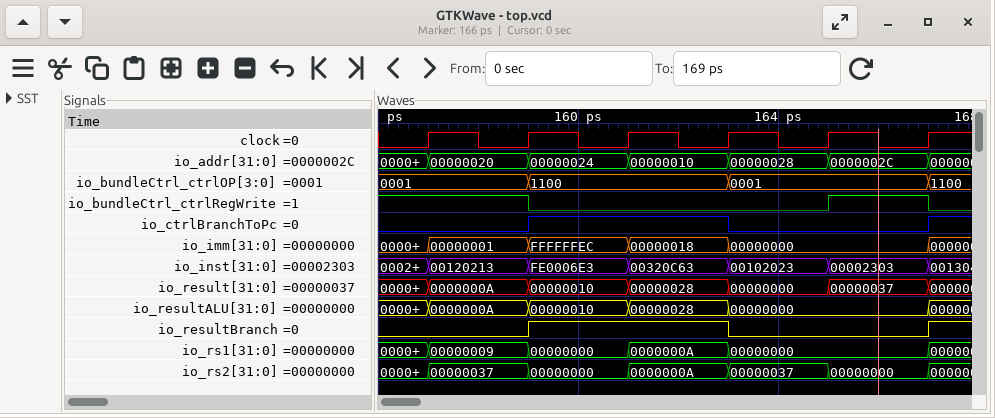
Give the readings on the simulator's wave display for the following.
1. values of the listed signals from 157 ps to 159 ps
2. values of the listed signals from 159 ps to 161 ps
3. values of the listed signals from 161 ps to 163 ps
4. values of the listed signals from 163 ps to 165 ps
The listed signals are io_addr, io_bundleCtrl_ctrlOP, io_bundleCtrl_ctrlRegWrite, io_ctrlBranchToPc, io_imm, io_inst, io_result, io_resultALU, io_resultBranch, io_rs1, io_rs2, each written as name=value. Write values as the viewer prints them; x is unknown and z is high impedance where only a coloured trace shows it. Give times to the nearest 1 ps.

io_addr=00000020, io_bundleCtrl_ctrlOP=0001, io_bundleCtrl_ctrlRegWrite=1, io_ctrlBranchToPc=0, io_imm=00000001, io_inst=00120213, io_result=0000000A, io_resultALU=0000000A, io_resultBranch=0, io_rs1=00000009, io_rs2=00000037
io_addr=00000024, io_bundleCtrl_ctrlOP=1100, io_bundleCtrl_ctrlRegWrite=0, io_ctrlBranchToPc=1, io_imm=FFFFFFEC, io_inst=FE0006E3, io_result=00000010, io_resultALU=00000010, io_resultBranch=1, io_rs1=00000000, io_rs2=00000000
io_addr=00000010, io_bundleCtrl_ctrlOP=1100, io_bundleCtrl_ctrlRegWrite=0, io_ctrlBranchToPc=1, io_imm=00000018, io_inst=00320C63, io_result=00000028, io_resultALU=00000028, io_resultBranch=1, io_rs1=0000000A, io_rs2=0000000A
io_addr=00000028, io_bundleCtrl_ctrlOP=0001, io_bundleCtrl_ctrlRegWrite=0, io_ctrlBranchToPc=0, io_imm=00000000, io_inst=00102023, io_result=00000000, io_resultALU=00000000, io_resultBranch=0, io_rs1=00000000, io_rs2=00000037
